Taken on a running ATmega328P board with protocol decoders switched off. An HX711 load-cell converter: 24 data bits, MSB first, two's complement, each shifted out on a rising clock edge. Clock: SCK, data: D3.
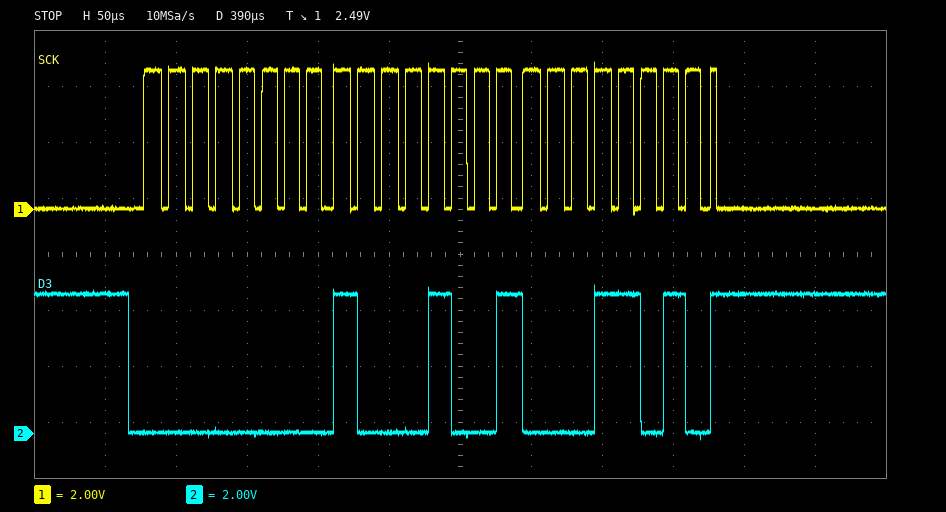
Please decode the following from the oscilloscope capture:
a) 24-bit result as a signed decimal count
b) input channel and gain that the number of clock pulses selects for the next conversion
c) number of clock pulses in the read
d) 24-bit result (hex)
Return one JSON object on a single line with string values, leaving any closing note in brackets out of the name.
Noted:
{"24-bit result as a signed decimal count": "35098", "input channel and gain that the number of clock pulses selects for the next conversion": "channel A, gain 128", "number of clock pulses in the read": "25", "24-bit result": "0x00891A"}
